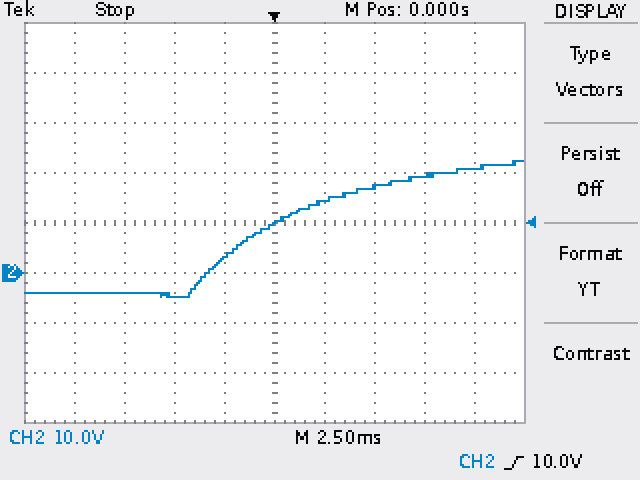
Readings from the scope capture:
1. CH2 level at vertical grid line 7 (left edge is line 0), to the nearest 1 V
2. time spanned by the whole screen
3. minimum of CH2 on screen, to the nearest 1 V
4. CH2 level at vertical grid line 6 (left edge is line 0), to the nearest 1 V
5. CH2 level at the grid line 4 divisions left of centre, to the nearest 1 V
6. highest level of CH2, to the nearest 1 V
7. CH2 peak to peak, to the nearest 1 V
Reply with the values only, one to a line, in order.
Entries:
17 V
25 ms
-5 V
14 V
-4 V
22 V
27 V
